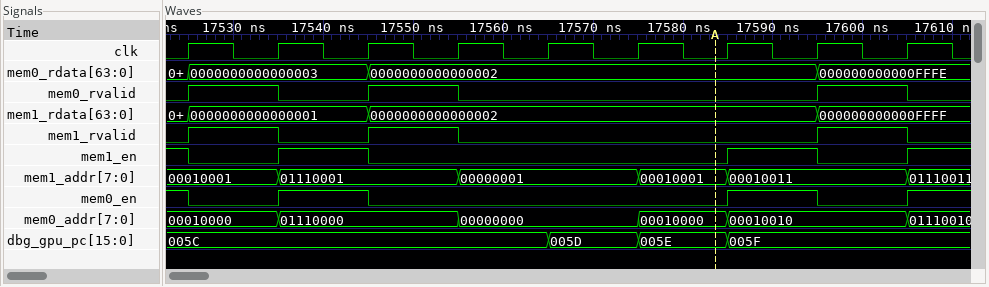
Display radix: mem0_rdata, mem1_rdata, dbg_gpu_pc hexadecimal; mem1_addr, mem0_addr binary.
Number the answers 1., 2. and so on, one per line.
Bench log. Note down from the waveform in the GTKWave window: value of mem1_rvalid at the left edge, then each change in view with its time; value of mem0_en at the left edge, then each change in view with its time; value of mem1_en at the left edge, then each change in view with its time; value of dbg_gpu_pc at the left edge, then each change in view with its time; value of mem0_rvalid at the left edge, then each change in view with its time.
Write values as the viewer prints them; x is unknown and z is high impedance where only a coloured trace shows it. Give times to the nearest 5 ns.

1. 0, 1 at 17525 ns, 0 at 17535 ns, 1 at 17545 ns, 0 at 17555 ns, 1 at 17595 ns, 0 at 17605 ns
2. 1, 0 at 17525 ns, 1 at 17535 ns, 0 at 17545 ns, 1 at 17585 ns, 0 at 17595 ns, 1 at 17605 ns
3. 1, 0 at 17525 ns, 1 at 17535 ns, 0 at 17545 ns, 1 at 17585 ns, 0 at 17595 ns, 1 at 17605 ns
4. 005C, 005D at 17565 ns, 005E at 17575 ns, 005F at 17585 ns
5. 0, 1 at 17525 ns, 0 at 17535 ns, 1 at 17545 ns, 0 at 17555 ns, 1 at 17595 ns, 0 at 17605 ns
